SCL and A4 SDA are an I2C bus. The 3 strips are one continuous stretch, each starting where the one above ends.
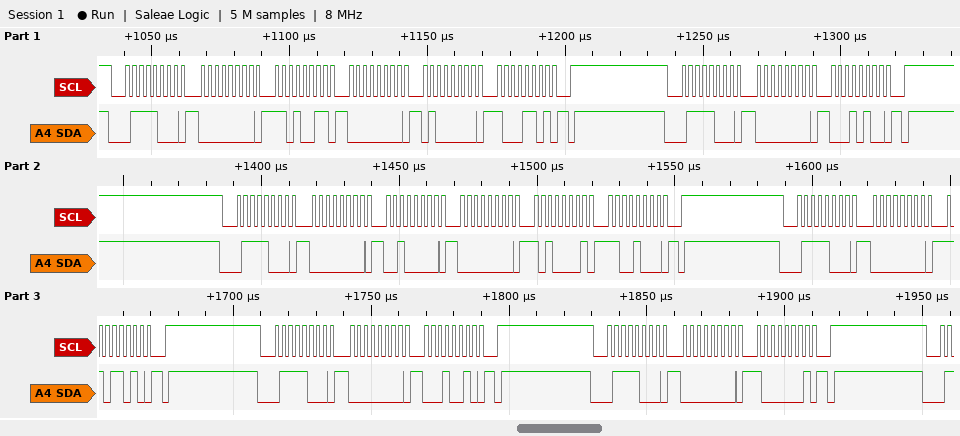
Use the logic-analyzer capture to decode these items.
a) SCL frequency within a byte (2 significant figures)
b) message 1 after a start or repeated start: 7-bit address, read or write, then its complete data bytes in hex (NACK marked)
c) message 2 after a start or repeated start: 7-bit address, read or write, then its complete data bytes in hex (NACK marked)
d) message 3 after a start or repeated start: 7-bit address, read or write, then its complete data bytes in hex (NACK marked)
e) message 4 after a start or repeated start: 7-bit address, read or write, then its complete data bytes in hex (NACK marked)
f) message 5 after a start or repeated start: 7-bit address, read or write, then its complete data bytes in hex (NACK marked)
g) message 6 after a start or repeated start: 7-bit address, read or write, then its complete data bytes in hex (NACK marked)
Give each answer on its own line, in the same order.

400 kHz
0x3C write: 00 D3 00 40 8D
0x3C write: 00 14
0x3C write: 00 20 00 A1 C8
0x3C write: 00 DA
0x3C write: 00 12
0x3C write: 00 81
